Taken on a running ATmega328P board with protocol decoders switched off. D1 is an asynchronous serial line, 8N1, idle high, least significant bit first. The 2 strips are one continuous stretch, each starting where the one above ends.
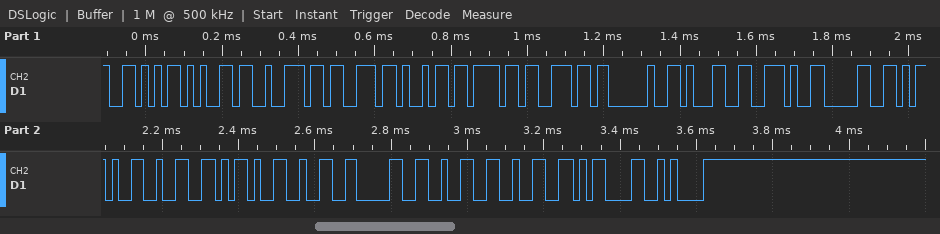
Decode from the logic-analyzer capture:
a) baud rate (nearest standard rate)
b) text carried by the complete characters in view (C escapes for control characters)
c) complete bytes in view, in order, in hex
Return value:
57600 baud
"Version 1.0-2-2022\r\n"
56 65 72 73 69 6F 6E 20 31 2E 30 2D 32 2D 32 30 32 32 0D 0A
